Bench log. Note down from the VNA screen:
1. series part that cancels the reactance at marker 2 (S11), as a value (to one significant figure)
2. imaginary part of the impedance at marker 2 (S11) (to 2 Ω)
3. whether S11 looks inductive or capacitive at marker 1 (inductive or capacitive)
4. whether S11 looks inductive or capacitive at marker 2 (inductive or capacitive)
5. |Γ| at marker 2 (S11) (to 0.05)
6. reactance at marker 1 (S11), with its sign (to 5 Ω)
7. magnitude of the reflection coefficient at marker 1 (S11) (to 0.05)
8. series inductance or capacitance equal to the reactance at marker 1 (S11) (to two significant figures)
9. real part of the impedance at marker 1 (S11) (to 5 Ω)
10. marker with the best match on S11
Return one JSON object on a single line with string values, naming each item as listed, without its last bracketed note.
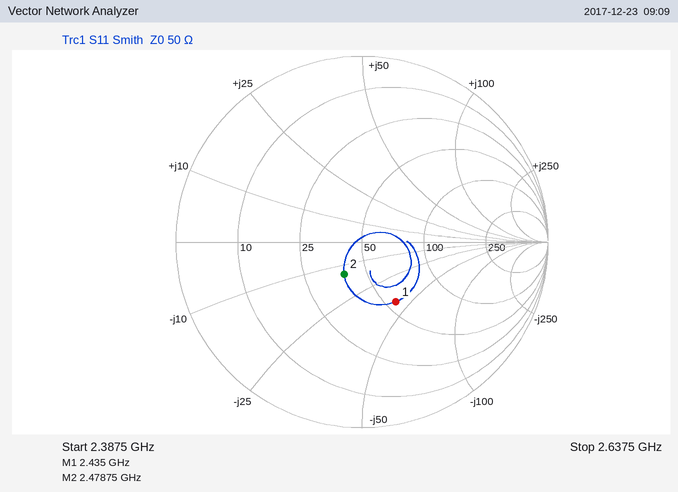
{"series part that cancels the reactance at marker 2 (S11), as a value": "900 pH", "imaginary part of the impedance at marker 2 (S11)": "-14 Ω", "whether S11 looks inductive or capacitive at marker 1": "capacitive", "whether S11 looks inductive or capacitive at marker 2": "capacitive", "|Γ| at marker 2 (S11)": "0.20", "reactance at marker 1 (S11), with its sign": "-40 Ω", "magnitude of the reflection coefficient at marker 1 (S11)": "0.35", "series inductance or capacitance equal to the reactance at marker 1 (S11)": "1.6 pF", "real part of the impedance at marker 1 (S11)": "55 Ω", "marker with the best match on S11": "marker 2"}
